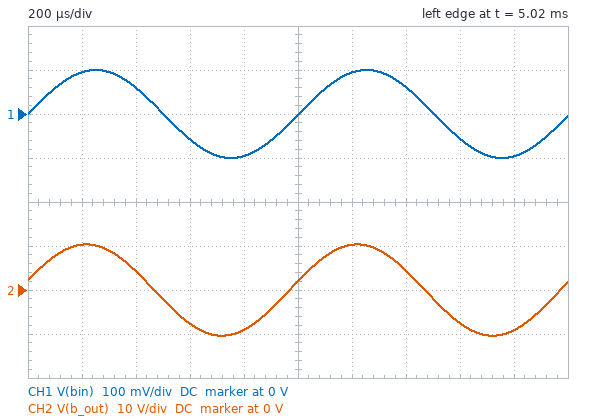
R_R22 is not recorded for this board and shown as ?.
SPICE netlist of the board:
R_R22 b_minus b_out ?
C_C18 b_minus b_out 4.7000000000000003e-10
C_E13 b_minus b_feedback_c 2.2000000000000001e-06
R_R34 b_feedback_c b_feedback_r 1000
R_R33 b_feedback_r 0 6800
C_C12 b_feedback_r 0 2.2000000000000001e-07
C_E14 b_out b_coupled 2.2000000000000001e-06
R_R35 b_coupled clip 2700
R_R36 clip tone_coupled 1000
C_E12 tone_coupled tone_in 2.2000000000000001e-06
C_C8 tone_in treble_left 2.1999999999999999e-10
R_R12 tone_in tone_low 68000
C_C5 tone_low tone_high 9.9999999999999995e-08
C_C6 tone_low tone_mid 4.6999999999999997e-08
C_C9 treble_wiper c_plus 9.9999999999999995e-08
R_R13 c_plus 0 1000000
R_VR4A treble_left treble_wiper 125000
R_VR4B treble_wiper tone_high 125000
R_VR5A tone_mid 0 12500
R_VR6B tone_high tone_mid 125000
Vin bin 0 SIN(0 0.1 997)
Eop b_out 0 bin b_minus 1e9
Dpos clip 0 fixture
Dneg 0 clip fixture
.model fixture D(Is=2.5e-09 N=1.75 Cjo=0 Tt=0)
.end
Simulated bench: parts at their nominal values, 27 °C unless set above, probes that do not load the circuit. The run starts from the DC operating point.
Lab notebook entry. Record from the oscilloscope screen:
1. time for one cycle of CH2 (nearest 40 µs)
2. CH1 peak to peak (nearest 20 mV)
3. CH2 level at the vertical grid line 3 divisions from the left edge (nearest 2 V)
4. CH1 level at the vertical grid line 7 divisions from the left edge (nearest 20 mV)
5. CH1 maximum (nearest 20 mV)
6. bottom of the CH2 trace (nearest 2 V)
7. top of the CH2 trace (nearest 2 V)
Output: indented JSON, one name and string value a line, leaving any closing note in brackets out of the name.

{
  "time for one cycle of CH2": "1.00 ms",
  "CH1 peak to peak": "200 mV",
  "CH2 level at the vertical grid line 3 divisions from the left edge": "-8 V",
  "CH1 level at the vertical grid line 7 divisions from the left edge": "60 mV",
  "CH1 maximum": "100 mV",
  "bottom of the CH2 trace": "-10 V",
  "top of the CH2 trace": "10 V"
}
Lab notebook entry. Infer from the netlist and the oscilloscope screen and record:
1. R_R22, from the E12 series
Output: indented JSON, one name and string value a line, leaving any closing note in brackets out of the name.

{
  "R_R22, from the E12 series": "150 kΩ"
}
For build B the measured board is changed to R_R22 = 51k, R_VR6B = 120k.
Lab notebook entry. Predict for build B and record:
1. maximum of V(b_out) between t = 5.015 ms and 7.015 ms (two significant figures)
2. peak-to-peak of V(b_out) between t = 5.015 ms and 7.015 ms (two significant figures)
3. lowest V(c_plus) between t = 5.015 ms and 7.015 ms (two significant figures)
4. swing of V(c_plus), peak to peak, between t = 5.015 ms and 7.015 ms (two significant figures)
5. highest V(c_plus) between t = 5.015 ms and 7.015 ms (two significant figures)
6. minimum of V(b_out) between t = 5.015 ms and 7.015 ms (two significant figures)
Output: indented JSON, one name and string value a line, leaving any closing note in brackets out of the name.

{
  "maximum of V(b_out) between t = 5.015 ms and 7.015 ms": "3.9 V",
  "peak-to-peak of V(b_out) between t = 5.015 ms and 7.015 ms": "7.7 V",
  "lowest V(c_plus) between t = 5.015 ms and 7.015 ms": "-290 mV",
  "swing of V(c_plus), peak to peak, between t = 5.015 ms and 7.015 ms": "590 mV",
  "highest V(c_plus) between t = 5.015 ms and 7.015 ms": "290 mV",
  "minimum of V(b_out) between t = 5.015 ms and 7.015 ms": "-3.9 V"
}
